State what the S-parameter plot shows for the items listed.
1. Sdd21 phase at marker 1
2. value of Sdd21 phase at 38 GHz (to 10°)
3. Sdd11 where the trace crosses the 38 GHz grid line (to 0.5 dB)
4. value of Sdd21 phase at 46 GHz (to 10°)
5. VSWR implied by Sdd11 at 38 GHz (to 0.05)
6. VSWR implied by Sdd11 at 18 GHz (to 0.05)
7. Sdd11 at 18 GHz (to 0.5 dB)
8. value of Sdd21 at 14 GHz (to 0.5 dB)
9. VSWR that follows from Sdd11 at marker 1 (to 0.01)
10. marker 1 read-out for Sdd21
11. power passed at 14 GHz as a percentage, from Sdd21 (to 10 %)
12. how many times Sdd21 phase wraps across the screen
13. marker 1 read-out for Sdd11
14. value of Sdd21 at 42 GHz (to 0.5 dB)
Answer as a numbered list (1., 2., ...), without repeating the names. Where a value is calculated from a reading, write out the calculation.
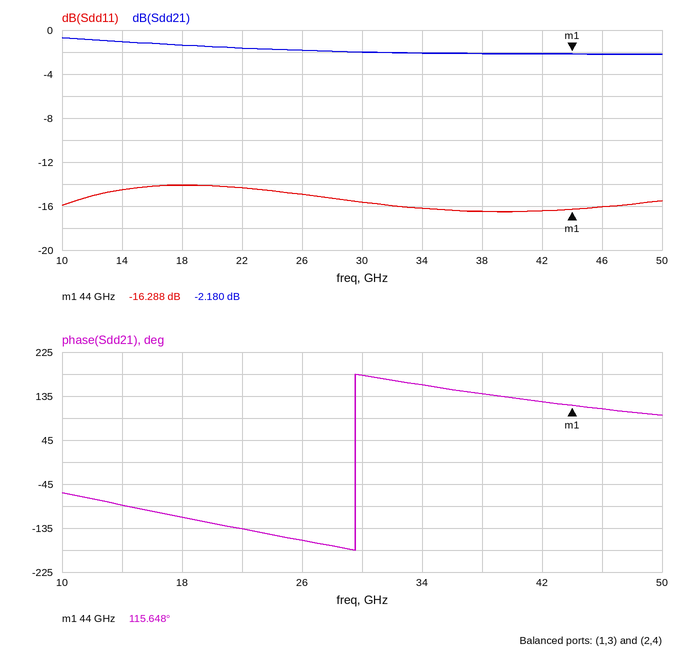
1. 115.648°
2. 140°
3. -16.5 dB
4. 110°
5. |Γ| = 10^(-16.5/20) = 0.1496; VSWR = (1 + 0.1496)/(1 − 0.1496) ≈ 1.35
6. |Γ| = 10^(-14/20) = 0.1995; VSWR = (1 + 0.1995)/(1 − 0.1995) ≈ 1.50
7. -14.0 dB
8. -1.0 dB
9. (1 + 0.1533)/(1 − 0.1533) ≈ 1.36
10. -2.180 dB
11. 10^(-1/10) ≈ 79.4 %, so 80 % to the nearest 10 %
12. 1
13. -16.288 dB
14. -2.0 dB
